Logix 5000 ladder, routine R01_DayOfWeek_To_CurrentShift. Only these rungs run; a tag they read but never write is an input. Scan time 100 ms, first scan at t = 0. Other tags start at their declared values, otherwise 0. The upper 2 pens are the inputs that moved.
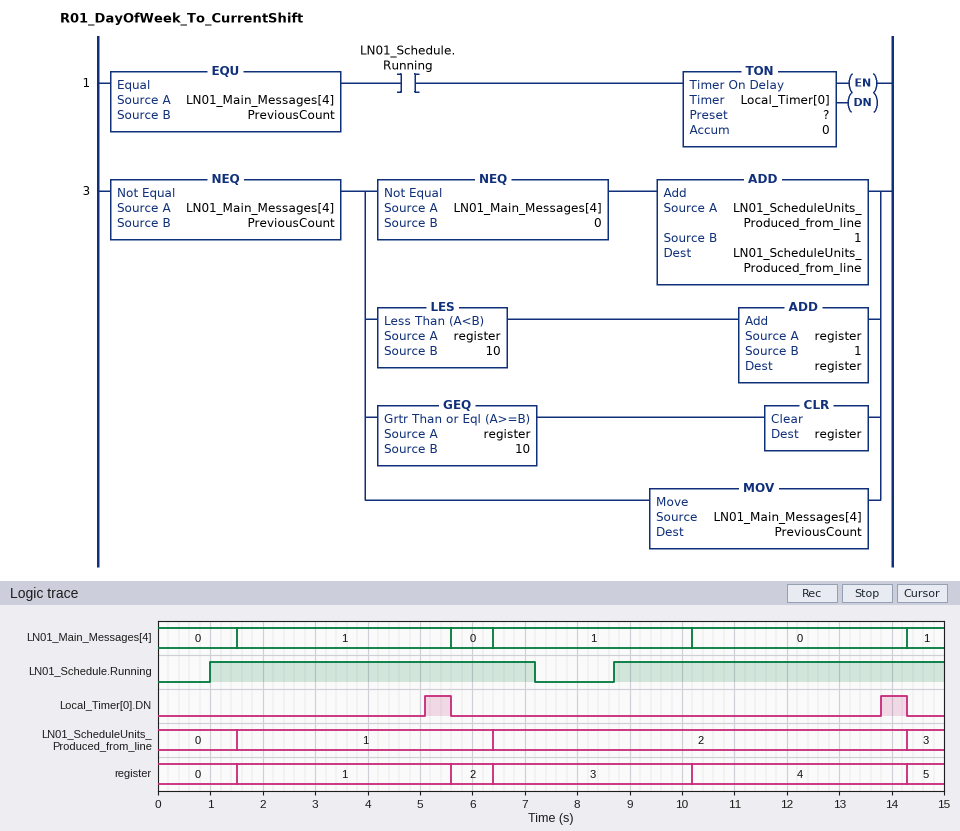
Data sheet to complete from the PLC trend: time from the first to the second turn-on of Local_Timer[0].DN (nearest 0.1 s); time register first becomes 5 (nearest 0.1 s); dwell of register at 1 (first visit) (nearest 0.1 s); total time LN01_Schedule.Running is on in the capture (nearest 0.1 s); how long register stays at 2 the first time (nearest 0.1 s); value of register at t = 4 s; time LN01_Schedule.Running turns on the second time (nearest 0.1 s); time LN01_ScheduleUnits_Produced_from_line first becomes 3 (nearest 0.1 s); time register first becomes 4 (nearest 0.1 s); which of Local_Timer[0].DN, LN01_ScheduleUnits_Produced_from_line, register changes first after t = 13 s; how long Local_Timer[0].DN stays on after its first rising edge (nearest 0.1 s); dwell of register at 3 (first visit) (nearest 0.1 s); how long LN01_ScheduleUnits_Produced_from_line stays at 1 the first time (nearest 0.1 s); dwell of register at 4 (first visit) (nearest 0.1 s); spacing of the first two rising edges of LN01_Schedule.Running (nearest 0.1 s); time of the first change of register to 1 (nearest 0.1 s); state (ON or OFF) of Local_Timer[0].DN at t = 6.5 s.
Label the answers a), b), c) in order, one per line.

a) 8.7 s
b) 14.3 s
c) 4.1 s
d) 12.5 s
e) 0.8 s
f) 1
g) 8.7 s
h) 14.3 s
i) 10.2 s
j) Local_Timer[0].DN
k) 0.5 s
l) 3.8 s
m) 4.9 s
n) 4.1 s
o) 7.7 s
p) 1.5 s
q) OFF
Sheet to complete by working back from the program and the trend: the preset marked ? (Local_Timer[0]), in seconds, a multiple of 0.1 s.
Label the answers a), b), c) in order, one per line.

a) 3.5 s
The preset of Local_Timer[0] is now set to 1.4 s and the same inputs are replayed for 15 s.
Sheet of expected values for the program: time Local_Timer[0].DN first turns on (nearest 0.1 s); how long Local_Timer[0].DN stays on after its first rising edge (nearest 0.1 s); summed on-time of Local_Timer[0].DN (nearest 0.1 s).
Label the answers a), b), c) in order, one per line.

a) 3.0 s
b) 2.6 s
c) 5.3 s
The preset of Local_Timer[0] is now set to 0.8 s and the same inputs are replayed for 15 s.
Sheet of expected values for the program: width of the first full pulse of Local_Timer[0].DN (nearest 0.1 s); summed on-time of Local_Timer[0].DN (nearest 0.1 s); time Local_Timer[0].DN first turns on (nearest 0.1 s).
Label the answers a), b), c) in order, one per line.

a) 3.2 s
b) 7.1 s
c) 2.4 s
